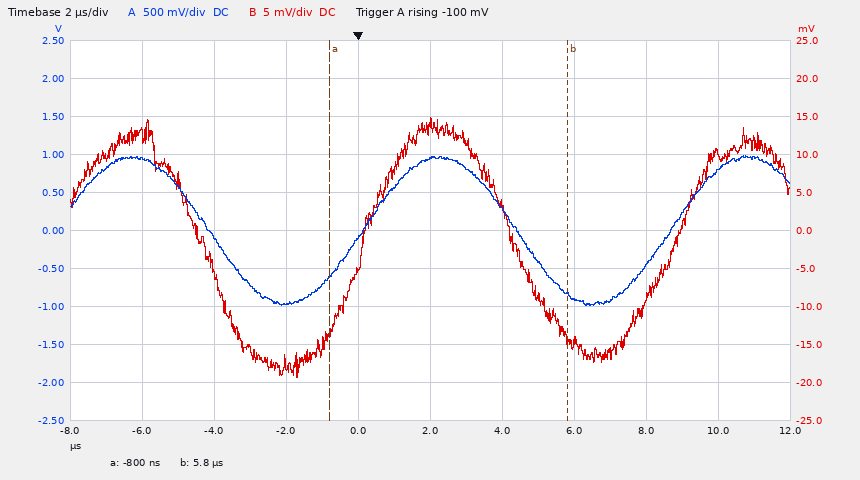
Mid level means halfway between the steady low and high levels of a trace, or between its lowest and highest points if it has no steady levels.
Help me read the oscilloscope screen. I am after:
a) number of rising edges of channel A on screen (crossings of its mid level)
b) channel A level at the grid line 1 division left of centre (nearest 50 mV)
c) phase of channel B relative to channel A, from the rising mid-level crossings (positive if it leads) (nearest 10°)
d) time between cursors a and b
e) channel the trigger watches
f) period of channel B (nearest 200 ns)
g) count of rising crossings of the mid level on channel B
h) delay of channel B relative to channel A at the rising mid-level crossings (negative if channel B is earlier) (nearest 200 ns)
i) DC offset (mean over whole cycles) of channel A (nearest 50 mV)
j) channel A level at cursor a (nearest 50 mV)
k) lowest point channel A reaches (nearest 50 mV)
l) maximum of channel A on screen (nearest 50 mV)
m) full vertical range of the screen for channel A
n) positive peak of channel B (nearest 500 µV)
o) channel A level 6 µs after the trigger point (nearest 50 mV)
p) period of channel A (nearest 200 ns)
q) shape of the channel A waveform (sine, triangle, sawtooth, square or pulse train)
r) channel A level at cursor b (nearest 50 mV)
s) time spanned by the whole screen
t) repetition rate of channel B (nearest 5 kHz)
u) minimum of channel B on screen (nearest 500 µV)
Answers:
2
-100 mV
0°
6.6 µs
channel A
8.6 µs
2
0.0 µs
0 mV
-600 mV
-1.00 V
1.00 V
5 V
15.0 mV
-900 mV
8.6 µs
sine
-850 mV
20 µs
115 kHz
-19.5 mV
